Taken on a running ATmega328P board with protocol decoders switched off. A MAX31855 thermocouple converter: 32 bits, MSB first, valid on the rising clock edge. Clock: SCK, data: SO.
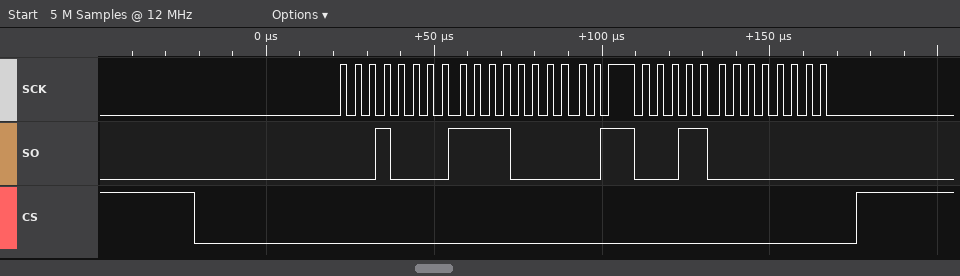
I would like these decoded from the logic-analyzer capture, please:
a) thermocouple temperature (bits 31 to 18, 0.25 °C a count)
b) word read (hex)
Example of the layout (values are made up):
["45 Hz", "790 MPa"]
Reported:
["271.00 °C", "0x10F02300"]
